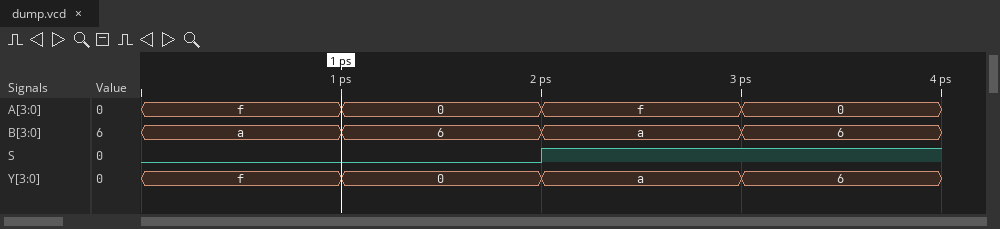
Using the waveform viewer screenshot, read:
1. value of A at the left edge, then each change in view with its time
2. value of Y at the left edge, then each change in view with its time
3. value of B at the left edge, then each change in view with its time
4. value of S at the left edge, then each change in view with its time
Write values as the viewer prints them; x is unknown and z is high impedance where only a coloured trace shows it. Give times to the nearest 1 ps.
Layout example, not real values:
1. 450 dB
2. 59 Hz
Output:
1. f, 0 at 1 ps, f at 2 ps, 0 at 3 ps
2. f, 0 at 1 ps, a at 2 ps, 6 at 3 ps
3. a, 6 at 1 ps, a at 2 ps, 6 at 3 ps
4. 0, 1 at 2 ps
